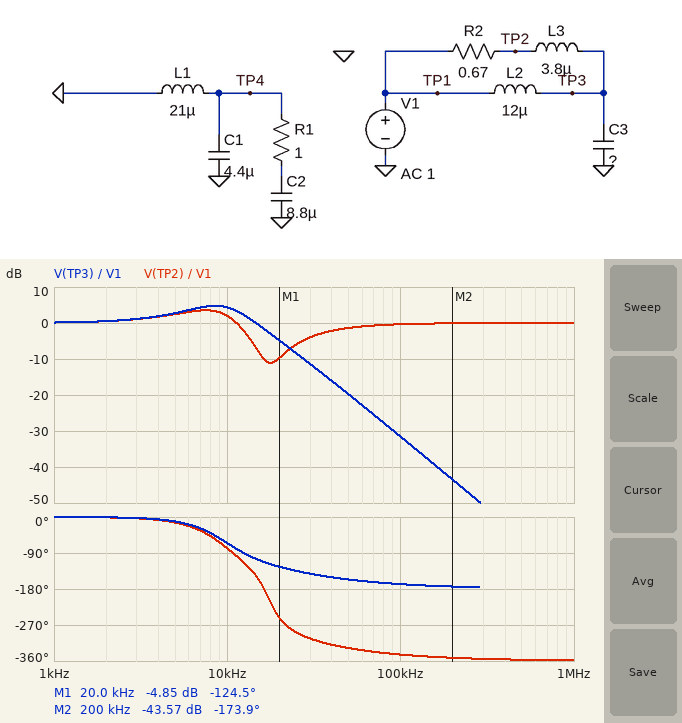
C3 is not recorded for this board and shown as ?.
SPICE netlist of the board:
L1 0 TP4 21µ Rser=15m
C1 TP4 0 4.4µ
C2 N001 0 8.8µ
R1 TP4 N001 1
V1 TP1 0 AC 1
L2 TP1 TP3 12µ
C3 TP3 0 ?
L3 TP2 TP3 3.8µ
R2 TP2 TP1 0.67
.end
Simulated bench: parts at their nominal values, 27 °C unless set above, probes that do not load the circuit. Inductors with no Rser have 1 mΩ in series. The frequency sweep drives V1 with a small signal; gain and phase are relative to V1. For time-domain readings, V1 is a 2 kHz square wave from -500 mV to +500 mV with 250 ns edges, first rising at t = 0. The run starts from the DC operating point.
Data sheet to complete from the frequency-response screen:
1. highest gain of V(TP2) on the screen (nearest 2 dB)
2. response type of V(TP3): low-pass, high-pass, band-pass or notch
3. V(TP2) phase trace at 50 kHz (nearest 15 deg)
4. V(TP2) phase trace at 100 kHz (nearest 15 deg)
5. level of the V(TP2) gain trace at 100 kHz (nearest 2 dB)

4 dB
low-pass
-330 deg
-345 deg
0 dB
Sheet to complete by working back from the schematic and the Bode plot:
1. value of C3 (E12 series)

33 µF
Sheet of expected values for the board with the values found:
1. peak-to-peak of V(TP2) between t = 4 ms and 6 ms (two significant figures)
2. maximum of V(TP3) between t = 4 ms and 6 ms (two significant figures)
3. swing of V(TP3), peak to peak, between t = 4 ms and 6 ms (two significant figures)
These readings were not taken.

1.8 V
930 mV
1.9 V
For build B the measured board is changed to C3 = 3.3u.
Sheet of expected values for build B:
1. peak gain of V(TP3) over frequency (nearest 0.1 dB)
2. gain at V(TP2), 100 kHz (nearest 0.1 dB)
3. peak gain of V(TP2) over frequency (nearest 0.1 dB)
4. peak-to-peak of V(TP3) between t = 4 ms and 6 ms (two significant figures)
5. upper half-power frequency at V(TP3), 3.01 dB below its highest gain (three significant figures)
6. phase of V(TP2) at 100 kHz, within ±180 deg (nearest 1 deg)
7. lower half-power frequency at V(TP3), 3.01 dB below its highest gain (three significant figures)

8.3 dB
-0.5 dB
0.5 dB
2.2 V
57.6 kHz
21 deg
35.6 kHz
